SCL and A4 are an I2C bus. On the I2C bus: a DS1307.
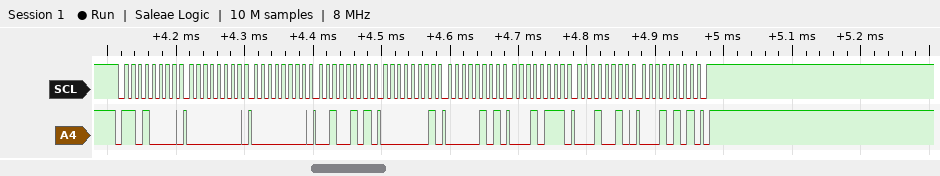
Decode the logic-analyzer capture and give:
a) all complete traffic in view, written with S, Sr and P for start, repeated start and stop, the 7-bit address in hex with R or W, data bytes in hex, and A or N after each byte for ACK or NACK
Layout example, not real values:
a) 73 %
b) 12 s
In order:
a) S 68W A 00 A 00 A 25 A 01 A 05 A 17 A 12 A 15 A P
